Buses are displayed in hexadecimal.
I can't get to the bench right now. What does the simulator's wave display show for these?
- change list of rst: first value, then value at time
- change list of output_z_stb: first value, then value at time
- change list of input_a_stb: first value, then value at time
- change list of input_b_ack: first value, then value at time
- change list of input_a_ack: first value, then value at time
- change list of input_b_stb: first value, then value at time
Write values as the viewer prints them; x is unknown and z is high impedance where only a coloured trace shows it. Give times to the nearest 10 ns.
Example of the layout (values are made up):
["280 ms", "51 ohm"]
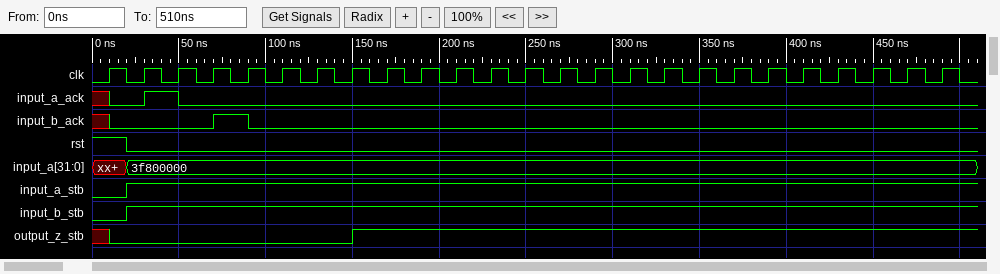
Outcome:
["1, 0 at 20 ns", "x, 0 at 10 ns, 1 at 150 ns", "0, 1 at 20 ns", "x, 0 at 10 ns, 1 at 70 ns, 0 at 90 ns", "x, 0 at 10 ns, 1 at 30 ns, 0 at 50 ns", "0, 1 at 20 ns"]
